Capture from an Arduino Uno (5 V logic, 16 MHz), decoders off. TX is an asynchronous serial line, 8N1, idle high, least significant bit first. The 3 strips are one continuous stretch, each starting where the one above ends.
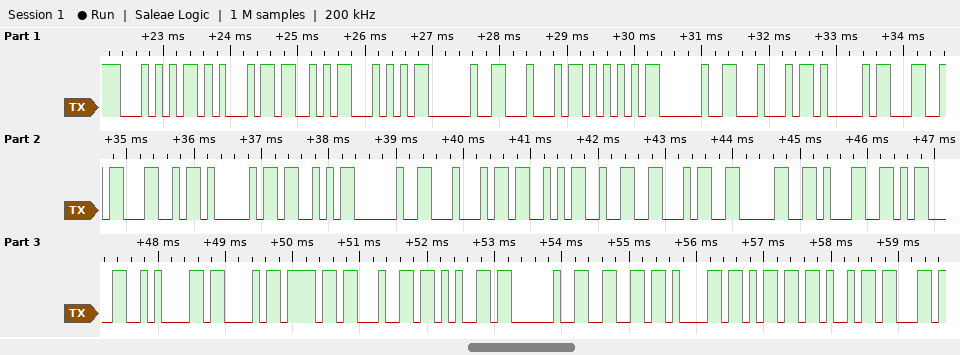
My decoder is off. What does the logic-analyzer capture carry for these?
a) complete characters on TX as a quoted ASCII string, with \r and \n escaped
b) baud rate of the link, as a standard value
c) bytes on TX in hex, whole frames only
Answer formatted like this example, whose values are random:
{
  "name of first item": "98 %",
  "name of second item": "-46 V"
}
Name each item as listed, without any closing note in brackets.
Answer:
{
  "complete characters on TX as a quoted ASCII string, with \\r and \\n escaped": "\"TEST DU DALLAS DS2401\\r\\nCode fami\"",
  "baud rate of the link, as a standard value": "9600 baud",
  "bytes on TX in hex, whole frames only": "54 45 53 54 20 44 55 20 44 41 4C 4C 41 53 20 44 53 32 34 30 31 0D 0A 43 6F 64 65 20 66 61 6D 69"
}
